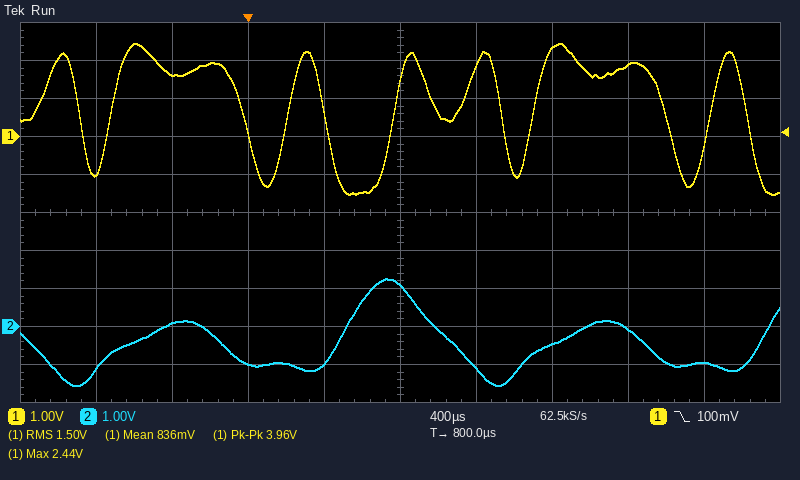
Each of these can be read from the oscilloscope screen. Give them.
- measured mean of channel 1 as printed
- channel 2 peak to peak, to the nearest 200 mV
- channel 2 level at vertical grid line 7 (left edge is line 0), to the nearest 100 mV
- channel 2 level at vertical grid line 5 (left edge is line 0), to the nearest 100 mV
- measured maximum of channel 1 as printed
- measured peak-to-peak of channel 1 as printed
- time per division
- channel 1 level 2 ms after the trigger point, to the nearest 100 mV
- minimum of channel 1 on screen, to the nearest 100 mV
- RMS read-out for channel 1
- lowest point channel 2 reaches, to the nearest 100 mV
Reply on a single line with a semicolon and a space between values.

836 mV; 2.8 V; -500 mV; 1.1 V; 2.44 V; 3.96 V; 400 µs; 1.9 V; -1.5 V; 1.50 V; -1.6 V
